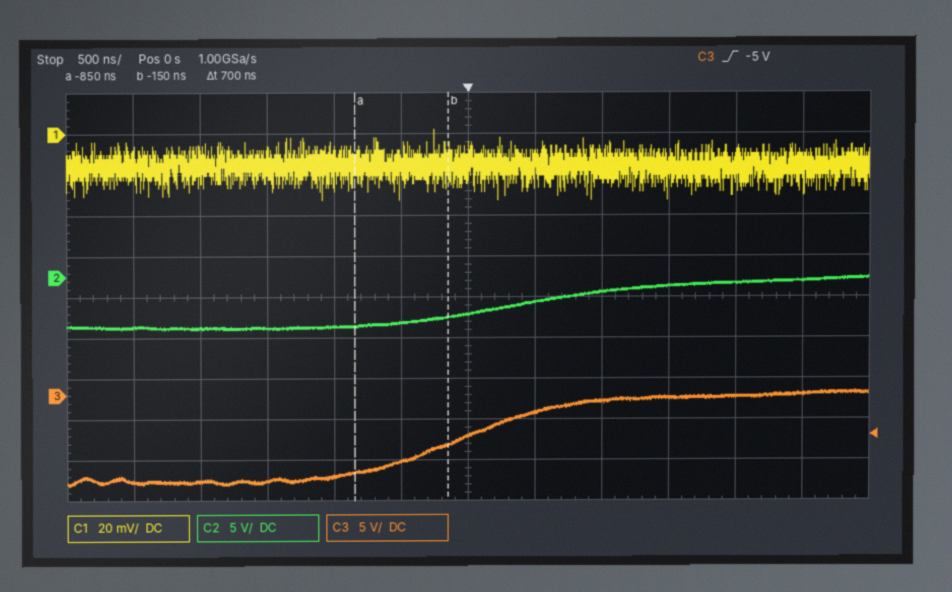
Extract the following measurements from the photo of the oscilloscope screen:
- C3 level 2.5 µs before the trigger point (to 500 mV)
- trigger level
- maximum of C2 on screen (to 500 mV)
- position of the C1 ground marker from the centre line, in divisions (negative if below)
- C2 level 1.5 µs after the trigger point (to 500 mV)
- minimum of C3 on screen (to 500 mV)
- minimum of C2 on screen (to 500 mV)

-10.5 V
-5 V
0.0 V
+4.0 div
-1.0 V
-11.0 V
-6.5 V
